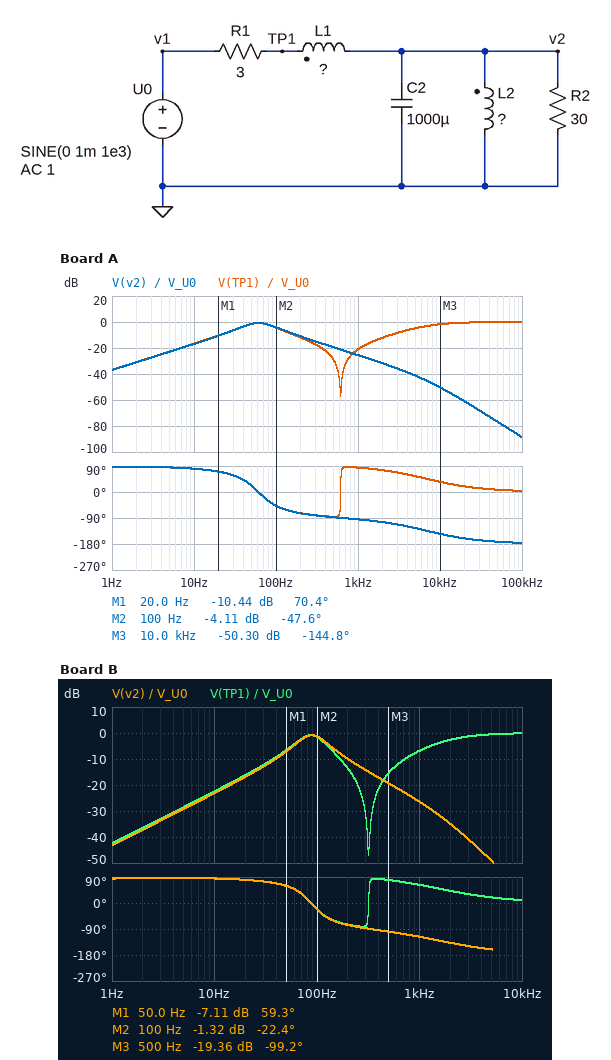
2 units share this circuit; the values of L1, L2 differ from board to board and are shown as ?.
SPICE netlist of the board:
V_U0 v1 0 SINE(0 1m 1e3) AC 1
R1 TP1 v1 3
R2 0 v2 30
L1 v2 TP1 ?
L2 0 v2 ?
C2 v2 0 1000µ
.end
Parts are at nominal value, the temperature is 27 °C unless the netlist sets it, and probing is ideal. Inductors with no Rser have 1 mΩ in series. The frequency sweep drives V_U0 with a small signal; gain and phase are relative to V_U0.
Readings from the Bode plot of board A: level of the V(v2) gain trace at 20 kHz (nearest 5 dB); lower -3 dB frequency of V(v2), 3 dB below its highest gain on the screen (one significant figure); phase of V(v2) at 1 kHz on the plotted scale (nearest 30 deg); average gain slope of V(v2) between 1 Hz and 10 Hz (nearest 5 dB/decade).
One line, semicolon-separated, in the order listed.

-60 dB; 40 Hz; -90 deg; 20 dB/decade
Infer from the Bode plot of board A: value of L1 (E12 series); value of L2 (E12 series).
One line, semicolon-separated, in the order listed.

68 µH; 6.8 mH
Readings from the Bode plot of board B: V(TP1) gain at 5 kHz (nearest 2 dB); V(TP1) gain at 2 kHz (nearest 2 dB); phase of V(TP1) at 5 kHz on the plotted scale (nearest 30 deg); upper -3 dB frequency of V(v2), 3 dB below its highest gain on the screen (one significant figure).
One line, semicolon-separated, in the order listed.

0 dB; -2 dB; 30 deg; 100 Hz
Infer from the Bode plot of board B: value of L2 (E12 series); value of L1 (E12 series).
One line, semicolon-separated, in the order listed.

3.3 mH; 270 µH
